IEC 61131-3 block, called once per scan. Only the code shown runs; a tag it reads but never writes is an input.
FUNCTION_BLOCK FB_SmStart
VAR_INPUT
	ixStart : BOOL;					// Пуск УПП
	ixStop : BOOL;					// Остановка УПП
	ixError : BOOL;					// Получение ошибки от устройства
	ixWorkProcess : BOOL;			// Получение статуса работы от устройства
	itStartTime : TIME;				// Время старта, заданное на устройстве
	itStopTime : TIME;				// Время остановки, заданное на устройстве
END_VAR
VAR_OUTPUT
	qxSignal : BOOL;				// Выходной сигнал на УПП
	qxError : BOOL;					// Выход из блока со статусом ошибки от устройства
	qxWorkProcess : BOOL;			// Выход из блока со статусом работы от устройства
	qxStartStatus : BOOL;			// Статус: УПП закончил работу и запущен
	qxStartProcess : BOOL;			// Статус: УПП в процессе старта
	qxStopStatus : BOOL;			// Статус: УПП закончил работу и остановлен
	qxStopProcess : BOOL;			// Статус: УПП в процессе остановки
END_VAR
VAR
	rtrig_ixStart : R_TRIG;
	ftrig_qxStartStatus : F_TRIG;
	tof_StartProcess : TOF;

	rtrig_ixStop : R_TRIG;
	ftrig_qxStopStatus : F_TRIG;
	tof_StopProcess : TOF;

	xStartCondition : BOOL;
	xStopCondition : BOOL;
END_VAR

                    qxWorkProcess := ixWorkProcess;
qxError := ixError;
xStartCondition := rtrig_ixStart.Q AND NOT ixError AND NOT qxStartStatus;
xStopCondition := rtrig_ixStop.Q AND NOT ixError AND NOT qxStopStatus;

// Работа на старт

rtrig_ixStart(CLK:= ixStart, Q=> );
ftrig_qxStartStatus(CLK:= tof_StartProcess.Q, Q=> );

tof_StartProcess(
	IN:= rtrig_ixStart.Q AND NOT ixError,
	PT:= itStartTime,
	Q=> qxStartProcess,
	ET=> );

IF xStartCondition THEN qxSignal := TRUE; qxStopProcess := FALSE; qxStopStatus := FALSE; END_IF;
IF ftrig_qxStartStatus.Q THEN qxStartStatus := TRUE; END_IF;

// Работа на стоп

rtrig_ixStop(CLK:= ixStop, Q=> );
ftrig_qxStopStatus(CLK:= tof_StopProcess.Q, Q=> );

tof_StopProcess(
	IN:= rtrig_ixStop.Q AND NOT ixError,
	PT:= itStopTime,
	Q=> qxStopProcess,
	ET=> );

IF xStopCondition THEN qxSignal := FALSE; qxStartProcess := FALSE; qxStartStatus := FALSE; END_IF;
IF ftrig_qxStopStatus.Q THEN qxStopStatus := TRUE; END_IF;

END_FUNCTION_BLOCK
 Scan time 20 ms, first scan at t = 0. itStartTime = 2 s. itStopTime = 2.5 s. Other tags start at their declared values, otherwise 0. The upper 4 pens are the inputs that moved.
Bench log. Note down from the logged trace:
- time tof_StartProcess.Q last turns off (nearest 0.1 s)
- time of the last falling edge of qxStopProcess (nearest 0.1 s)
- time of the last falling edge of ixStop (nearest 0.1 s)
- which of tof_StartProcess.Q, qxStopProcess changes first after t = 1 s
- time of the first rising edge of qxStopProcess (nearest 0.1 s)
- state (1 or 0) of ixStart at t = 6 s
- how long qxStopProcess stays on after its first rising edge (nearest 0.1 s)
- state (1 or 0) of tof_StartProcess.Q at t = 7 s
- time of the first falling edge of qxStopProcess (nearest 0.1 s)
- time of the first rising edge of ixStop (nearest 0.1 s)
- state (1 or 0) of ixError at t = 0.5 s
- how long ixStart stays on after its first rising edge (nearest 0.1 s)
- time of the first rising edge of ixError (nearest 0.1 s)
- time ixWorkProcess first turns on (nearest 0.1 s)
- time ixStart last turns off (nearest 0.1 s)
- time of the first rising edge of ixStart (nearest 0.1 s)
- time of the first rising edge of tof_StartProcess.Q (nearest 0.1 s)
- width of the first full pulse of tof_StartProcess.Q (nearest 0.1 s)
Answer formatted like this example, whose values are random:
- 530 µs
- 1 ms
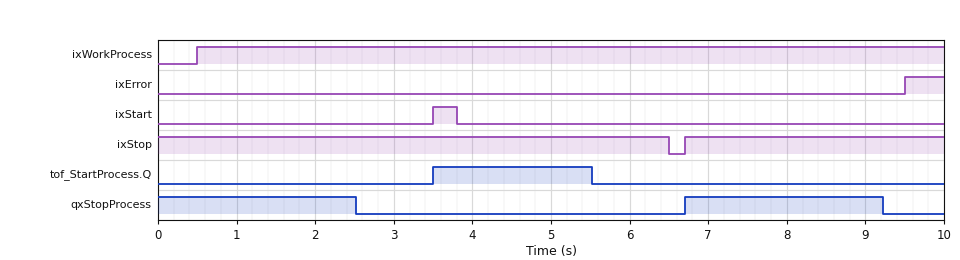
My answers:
- 5.5 s
- 9.2 s
- 6.5 s
- qxStopProcess
- 6.7 s
- 0
- 2.5 s
- 0
- 2.5 s
- 6.7 s
- 0
- 0.3 s
- 9.5 s
- 0.5 s
- 3.8 s
- 3.5 s
- 3.5 s
- 2.0 s
